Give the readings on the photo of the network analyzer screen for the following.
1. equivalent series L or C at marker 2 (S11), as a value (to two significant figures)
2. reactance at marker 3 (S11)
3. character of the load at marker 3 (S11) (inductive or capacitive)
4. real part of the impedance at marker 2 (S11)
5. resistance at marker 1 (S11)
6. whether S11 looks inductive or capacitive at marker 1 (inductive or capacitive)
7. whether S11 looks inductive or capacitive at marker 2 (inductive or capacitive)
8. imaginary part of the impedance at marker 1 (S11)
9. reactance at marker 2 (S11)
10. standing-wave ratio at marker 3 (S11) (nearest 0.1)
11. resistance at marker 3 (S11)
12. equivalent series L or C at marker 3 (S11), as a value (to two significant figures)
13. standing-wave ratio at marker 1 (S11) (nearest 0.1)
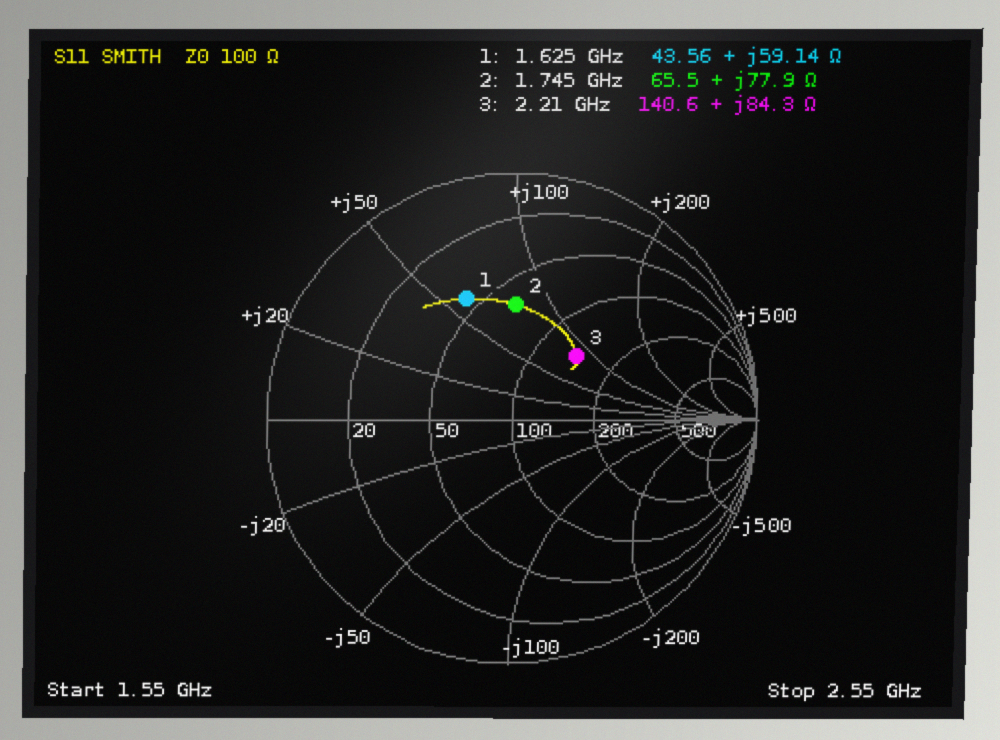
7.1 nH
+84.3 Ω
inductive
65.5 Ω
43.56 Ω
inductive
inductive
+59.14 Ω
+77.9 Ω
2.2
140.6 Ω
6.1 nH
3.2
